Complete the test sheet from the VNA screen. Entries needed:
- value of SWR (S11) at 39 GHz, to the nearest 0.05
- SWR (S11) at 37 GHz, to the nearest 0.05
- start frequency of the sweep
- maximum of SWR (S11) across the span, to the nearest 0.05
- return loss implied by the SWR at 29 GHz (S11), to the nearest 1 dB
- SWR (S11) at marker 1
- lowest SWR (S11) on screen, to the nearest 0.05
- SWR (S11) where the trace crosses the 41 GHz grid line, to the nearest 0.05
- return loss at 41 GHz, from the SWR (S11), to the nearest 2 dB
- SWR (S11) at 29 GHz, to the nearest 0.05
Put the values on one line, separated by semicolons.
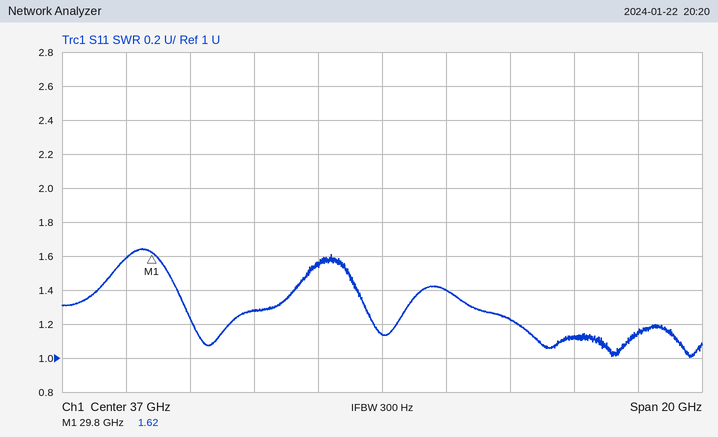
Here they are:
1.40; 1.15; 27 GHz; 1.65; 13 dB; 1.62; 1.00; 1.25; 20 dB; 1.60
